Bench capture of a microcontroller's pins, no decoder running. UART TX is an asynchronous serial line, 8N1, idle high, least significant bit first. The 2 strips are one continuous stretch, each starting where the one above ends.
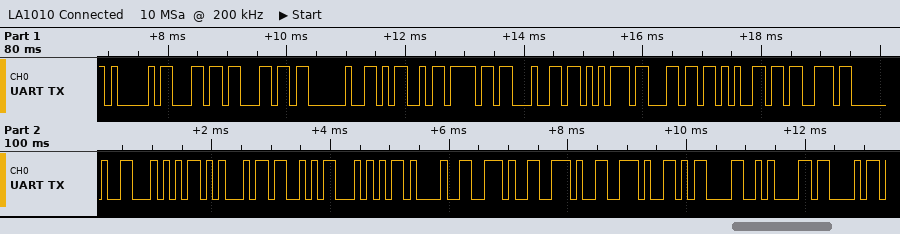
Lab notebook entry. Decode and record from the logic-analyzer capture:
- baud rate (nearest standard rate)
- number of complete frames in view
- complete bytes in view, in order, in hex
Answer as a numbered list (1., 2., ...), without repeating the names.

1. 9600 baud
2. 23
3. 0x41 0x6C 0x6C 0x20 0x4D 0x6F 0x64 0x75 0x6C 0x65 0x73 0x20 0x54 0x45 0x53 0x54 0x21 0x2E 0x2E 0x2E 0x0D 0x0A 0x43
